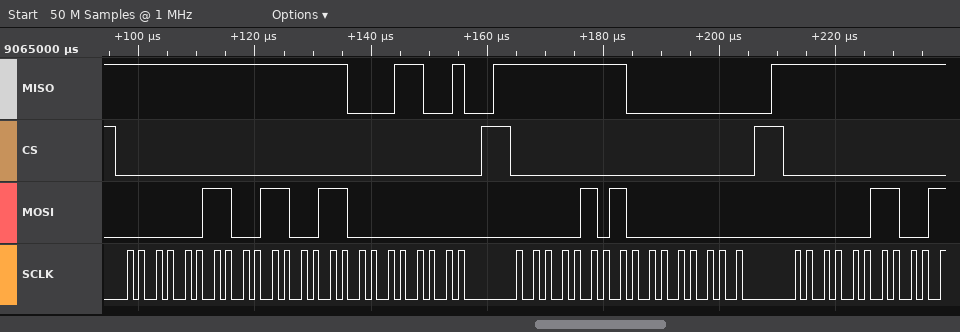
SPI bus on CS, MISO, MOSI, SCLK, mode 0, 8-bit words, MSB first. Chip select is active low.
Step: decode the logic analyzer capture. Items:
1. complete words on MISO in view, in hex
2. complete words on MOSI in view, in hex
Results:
FF, FF, 19, FF, 00, FF
03, 33, 00, 05, 00, 03
